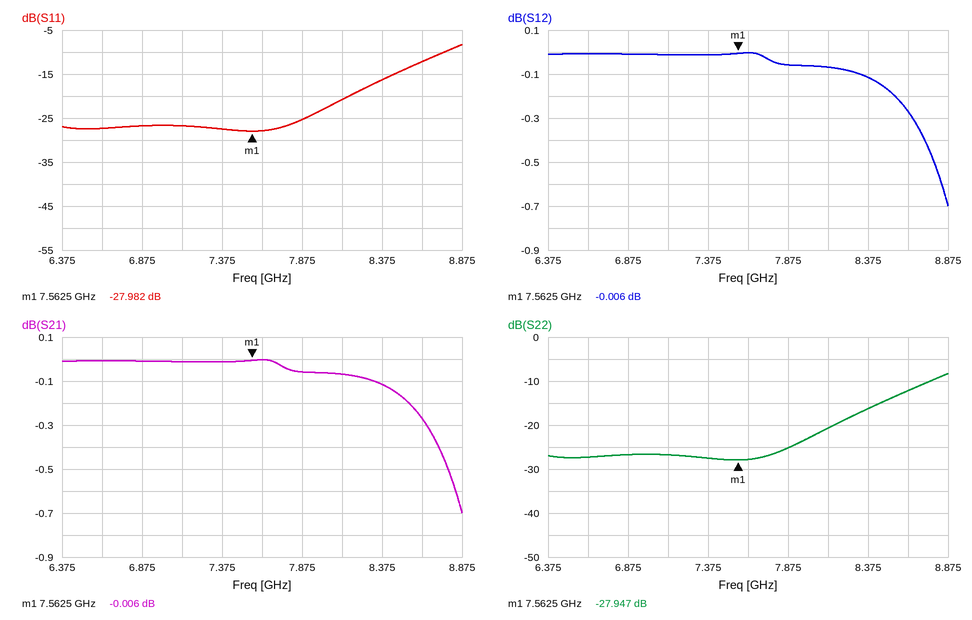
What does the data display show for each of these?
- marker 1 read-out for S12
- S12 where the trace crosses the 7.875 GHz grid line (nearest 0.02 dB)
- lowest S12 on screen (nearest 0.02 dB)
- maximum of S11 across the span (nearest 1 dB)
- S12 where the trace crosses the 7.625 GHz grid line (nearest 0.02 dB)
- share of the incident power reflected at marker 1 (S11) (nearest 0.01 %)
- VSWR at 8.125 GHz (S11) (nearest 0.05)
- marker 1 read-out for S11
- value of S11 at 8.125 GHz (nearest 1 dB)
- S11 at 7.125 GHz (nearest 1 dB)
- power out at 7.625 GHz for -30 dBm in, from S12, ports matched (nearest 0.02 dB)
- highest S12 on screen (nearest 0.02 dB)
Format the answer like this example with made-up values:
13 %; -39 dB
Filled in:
-0.006 dB; -0.06 dB; -0.70 dB; -8 dB; 0.00 dB; 0.16 %; 1.20; -27.982 dB; -21 dB; -27 dB; -30.00 dBm; 0.00 dB
